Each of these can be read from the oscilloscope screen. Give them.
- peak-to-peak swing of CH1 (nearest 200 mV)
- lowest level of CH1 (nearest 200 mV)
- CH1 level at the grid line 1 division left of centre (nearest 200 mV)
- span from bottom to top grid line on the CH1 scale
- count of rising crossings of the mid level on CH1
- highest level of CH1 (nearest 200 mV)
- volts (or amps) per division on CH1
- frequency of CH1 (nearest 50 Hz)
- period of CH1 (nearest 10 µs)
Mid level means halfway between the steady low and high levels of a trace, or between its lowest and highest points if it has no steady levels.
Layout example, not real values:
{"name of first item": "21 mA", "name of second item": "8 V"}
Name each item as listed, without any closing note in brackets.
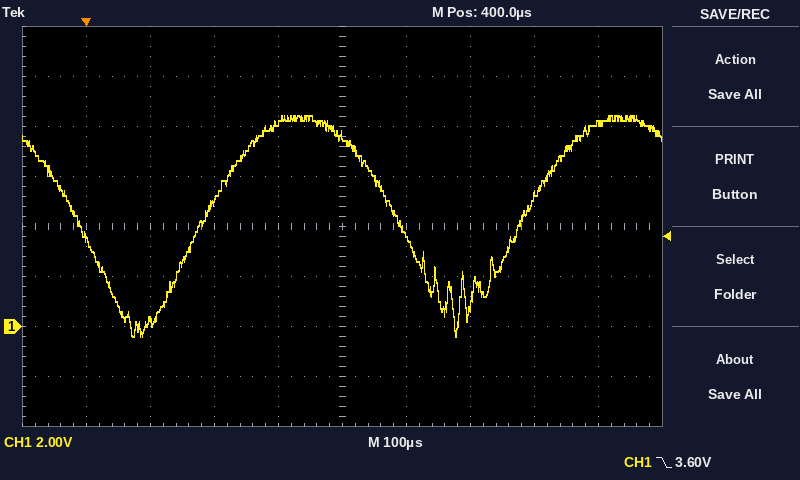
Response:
{"peak-to-peak swing of CH1": "8.8 V", "lowest level of CH1": "-400 mV", "CH1 level at the grid line 1 division left of centre": "8.2 V", "span from bottom to top grid line on the CH1 scale": "16 V", "count of rising crossings of the mid level on CH1": "2", "highest level of CH1": "8.4 V", "volts (or amps) per division on CH1": "2 V", "frequency of CH1": "2.00 kHz", "period of CH1": "500 µs"}
